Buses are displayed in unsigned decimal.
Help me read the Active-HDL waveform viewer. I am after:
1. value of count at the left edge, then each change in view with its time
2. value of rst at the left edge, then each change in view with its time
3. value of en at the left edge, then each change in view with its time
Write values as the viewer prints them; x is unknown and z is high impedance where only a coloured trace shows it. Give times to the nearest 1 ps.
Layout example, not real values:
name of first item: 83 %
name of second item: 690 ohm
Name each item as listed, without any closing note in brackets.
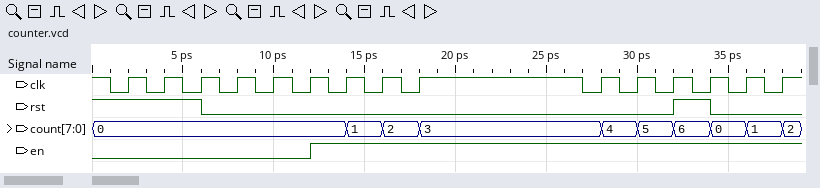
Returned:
value of count at the left edge, then each change in view with its time: 0, 1 at 14 ps, 2 at 16 ps, 3 at 18 ps, 4 at 28 ps, 5 at 30 ps, 6 at 32 ps, 0 at 34 ps, 1 at 36 ps, 2 at 38 ps
value of rst at the left edge, then each change in view with its time: 1, 0 at 6 ps, 1 at 32 ps, 0 at 34 ps
value of en at the left edge, then each change in view with its time: 0, 1 at 12 ps
